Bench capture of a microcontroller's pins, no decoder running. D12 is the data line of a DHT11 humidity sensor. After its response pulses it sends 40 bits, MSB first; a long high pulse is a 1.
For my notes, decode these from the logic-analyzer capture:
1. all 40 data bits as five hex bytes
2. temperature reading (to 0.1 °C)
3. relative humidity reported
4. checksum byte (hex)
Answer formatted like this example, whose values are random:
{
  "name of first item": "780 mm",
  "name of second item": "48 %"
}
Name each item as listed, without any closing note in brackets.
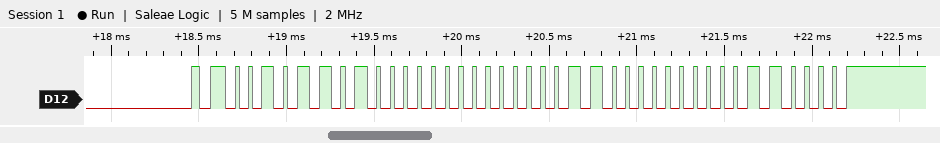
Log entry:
{
  "all 40 data bits as five hex bytes": "2D 00 03 00 30",
  "temperature reading": "3.0 °C",
  "relative humidity reported": "45 %",
  "checksum byte": "0x30"
}
